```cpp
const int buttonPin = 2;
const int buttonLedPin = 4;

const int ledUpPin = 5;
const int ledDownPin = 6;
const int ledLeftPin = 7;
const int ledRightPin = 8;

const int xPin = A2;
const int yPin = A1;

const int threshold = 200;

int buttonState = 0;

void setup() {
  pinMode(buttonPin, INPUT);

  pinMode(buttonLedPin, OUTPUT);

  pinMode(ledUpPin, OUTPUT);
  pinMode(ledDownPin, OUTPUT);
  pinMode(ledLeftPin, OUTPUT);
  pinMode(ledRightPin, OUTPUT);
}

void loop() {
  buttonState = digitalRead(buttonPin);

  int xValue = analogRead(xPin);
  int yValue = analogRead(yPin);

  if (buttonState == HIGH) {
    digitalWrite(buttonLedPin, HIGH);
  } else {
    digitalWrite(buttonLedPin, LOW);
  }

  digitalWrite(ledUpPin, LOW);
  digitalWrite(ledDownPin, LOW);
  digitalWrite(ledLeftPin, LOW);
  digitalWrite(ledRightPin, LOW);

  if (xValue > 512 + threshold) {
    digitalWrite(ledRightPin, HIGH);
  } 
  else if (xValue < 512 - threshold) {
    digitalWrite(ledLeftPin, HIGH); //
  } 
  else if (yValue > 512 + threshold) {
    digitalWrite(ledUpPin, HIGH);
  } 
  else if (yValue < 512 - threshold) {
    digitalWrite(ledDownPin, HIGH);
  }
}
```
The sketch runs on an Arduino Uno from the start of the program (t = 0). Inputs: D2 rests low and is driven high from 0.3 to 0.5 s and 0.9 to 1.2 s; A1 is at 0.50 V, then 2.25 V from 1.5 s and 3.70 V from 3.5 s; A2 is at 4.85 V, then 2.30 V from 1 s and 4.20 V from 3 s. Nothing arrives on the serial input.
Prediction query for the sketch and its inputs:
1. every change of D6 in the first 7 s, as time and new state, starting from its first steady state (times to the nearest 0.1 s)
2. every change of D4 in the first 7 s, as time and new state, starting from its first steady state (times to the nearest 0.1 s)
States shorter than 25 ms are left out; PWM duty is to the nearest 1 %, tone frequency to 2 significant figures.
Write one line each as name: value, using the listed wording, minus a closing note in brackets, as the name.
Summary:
every change of D6 in the first 7 s, as time and new state, starting from its first steady state: 0 s low; 1 s tone 4000 Hz; 1.5 s low
every change of D4 in the first 7 s, as time and new state, starting from its first steady state: 0 s low; 0.3 s high; 0.5 s low; 0.9 s high; 1.2 s low
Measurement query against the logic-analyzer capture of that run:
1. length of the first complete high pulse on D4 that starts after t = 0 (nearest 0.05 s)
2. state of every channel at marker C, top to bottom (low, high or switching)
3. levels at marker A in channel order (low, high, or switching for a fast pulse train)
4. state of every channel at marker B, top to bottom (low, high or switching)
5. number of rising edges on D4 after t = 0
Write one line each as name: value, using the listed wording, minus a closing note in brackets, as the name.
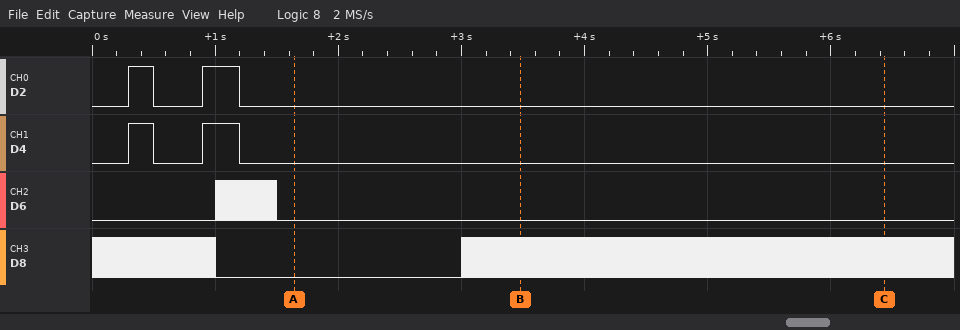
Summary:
length of the first complete high pulse on D4 that starts after t = 0: 0.20 s
state of every channel at marker C, top to bottom: D2 low, D4 low, D6 low, D8 switching
levels at marker A in channel order: D2 low, D4 low, D6 low, D8 low
state of every channel at marker B, top to bottom: D2 low, D4 low, D6 low, D8 switching
number of rising edges on D4 after t = 0: 2
